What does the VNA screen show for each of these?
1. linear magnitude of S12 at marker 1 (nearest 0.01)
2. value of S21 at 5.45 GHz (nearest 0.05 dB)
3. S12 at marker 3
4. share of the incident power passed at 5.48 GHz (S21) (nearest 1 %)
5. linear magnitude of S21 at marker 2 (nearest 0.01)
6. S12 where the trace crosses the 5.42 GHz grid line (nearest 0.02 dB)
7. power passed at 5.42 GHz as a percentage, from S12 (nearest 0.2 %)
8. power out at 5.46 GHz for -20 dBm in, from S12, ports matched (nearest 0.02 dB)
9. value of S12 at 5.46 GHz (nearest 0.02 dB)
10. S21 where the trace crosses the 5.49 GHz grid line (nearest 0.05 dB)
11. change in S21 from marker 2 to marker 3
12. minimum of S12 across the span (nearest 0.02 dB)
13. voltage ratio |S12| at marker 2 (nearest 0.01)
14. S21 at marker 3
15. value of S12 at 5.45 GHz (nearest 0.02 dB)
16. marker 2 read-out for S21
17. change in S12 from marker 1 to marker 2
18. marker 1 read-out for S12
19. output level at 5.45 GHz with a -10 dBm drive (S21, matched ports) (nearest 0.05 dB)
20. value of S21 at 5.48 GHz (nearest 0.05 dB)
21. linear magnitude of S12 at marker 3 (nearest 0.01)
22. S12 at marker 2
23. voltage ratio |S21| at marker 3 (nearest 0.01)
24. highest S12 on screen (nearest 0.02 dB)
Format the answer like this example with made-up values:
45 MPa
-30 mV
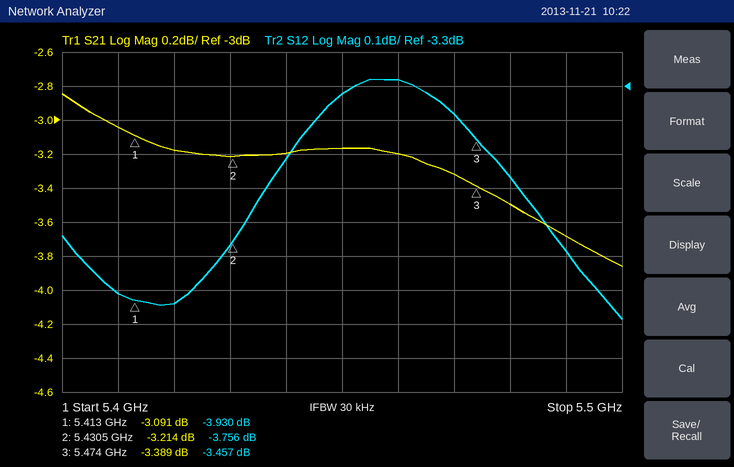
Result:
0.64
-3.15 dB
-3.457 dB
45 %
0.69
-3.94 dB
40.4 %
-23.28 dBm
-3.28 dB
-3.70 dB
-0.175 dB
-3.98 dB
0.65
-3.389 dB
-3.32 dB
-3.214 dB
0.174 dB
-3.930 dB
-13.15 dBm
-3.50 dB
0.67
-3.756 dB
0.68
-3.28 dB
